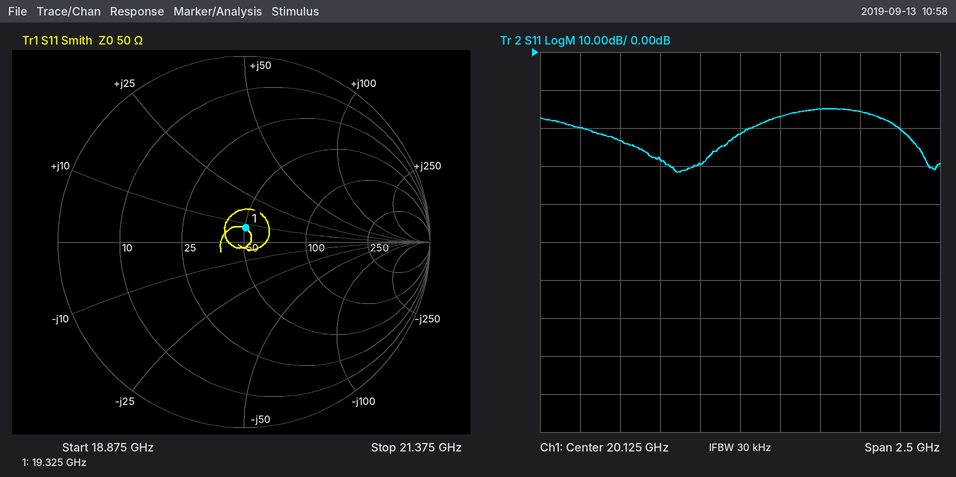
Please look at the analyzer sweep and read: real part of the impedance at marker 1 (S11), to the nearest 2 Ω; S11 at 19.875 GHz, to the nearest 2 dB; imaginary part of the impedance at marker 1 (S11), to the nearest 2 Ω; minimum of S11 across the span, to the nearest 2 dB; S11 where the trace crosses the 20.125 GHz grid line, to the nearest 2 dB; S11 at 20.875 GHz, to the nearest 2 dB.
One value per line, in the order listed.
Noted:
50 Ω
-30 dB
+8 Ω
-32 dB
-22 dB
-16 dB
